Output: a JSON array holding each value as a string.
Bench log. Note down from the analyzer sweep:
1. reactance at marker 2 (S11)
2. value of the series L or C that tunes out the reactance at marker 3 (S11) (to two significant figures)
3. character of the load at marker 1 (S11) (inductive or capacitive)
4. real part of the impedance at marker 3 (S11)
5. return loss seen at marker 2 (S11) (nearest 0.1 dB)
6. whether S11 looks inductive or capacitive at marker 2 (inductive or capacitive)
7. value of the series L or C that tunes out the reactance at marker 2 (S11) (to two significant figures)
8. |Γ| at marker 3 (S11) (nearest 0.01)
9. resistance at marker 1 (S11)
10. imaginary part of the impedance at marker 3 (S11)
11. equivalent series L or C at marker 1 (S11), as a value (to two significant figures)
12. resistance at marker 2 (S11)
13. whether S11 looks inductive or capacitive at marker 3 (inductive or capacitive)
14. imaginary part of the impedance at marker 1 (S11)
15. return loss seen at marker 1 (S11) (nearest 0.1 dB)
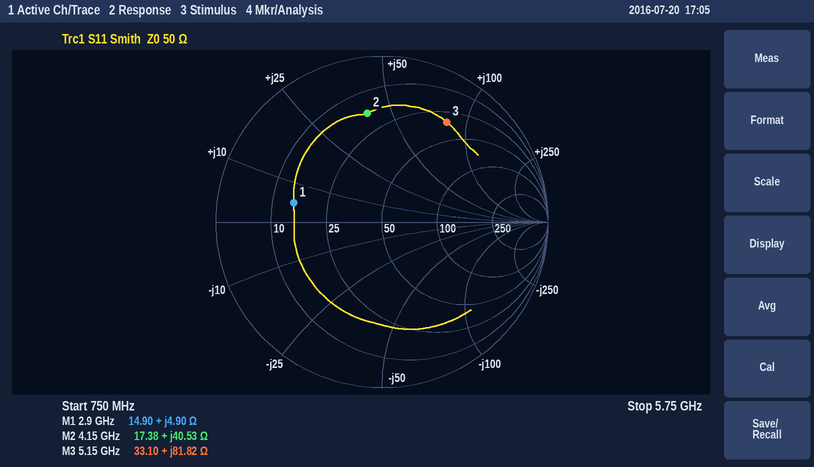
["+40.53 Ω", "380 fF", "inductive", "33.10 Ω", "3.6 dB", "inductive", "950 fF", "0.72", "14.90 Ω", "+81.82 Ω", "270 pH", "17.38 Ω", "inductive", "+4.90 Ω", "5.3 dB"]
